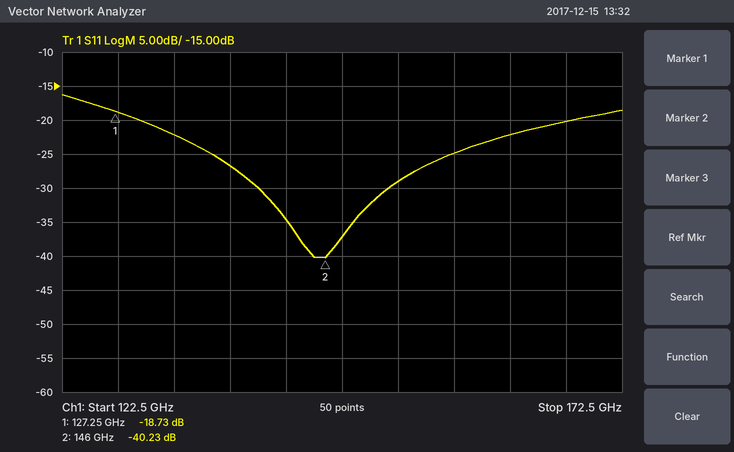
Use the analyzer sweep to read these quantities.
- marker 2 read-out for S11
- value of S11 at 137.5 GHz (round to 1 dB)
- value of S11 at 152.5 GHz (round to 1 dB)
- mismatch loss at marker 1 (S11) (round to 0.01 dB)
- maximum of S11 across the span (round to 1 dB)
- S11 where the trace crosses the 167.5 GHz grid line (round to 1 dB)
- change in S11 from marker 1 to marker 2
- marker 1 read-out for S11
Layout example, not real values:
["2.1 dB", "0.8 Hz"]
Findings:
["-40.23 dB", "-27 dB", "-29 dB", "0.06 dB", "-16 dB", "-20 dB", "-21.50 dB", "-18.73 dB"]
